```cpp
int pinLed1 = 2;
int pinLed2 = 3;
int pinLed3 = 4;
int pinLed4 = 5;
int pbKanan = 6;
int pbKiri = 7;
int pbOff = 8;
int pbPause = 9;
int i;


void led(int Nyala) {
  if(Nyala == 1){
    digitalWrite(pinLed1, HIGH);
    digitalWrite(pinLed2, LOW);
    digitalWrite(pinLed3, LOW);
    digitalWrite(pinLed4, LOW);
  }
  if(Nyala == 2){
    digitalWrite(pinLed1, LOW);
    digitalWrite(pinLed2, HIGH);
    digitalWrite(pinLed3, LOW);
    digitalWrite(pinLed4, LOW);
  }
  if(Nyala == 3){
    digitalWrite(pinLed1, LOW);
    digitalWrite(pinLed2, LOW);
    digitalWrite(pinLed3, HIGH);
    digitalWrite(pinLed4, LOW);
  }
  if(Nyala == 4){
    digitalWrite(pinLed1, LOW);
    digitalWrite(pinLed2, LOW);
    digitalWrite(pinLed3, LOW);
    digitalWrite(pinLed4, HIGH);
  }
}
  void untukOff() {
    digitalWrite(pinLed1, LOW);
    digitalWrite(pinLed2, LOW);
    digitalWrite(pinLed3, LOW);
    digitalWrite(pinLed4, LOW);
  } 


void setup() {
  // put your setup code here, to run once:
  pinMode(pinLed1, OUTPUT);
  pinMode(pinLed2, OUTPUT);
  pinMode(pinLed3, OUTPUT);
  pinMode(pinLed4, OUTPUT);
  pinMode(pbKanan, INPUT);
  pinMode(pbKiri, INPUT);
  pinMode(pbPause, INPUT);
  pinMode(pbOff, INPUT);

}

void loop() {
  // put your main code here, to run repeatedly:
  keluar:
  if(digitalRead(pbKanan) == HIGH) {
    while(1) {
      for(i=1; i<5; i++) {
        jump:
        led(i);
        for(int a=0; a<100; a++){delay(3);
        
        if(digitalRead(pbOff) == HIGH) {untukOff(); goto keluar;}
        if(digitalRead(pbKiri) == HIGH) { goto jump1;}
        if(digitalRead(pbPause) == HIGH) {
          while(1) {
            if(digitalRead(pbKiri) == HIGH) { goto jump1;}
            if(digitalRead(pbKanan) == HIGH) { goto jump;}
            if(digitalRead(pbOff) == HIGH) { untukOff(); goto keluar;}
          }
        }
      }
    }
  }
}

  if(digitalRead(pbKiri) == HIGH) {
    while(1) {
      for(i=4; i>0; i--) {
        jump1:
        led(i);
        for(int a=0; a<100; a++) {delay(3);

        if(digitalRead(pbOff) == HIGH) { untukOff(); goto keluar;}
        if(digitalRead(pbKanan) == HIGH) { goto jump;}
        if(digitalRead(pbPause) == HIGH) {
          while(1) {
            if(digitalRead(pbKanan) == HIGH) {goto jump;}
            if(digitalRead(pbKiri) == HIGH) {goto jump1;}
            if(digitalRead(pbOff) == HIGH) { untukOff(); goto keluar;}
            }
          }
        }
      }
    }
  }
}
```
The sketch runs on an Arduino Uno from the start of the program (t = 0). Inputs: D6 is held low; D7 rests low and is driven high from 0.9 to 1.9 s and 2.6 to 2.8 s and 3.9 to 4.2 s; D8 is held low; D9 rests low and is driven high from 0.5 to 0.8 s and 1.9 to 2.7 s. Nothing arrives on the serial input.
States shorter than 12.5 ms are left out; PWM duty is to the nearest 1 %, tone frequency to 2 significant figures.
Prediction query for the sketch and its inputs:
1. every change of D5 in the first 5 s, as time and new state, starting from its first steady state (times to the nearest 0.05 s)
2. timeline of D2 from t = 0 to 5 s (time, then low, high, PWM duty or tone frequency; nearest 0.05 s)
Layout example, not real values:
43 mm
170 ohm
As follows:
0 s low; 0.9 s high; 1.2 s low; 3 s high; 3.3 s low; 4.2 s high; 4.5 s low
0 s low; 1.8 s high; 3 s low; 3.9 s high; 4.2 s low
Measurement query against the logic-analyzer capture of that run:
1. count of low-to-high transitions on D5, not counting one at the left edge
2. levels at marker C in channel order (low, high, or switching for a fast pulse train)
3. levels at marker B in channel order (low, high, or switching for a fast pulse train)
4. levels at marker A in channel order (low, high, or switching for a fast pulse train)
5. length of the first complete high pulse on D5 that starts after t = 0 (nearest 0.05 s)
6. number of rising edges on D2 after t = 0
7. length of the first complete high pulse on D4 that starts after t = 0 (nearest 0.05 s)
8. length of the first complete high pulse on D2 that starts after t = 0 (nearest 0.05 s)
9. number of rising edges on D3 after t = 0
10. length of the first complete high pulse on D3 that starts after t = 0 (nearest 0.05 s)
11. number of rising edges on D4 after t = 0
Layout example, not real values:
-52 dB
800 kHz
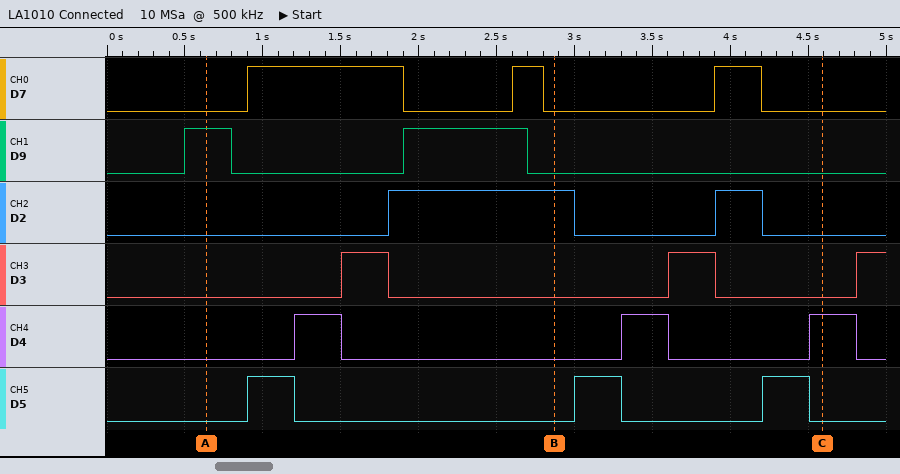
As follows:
3
D7 low, D9 low, D2 low, D3 low, D4 high, D5 low
D7 low, D9 low, D2 high, D3 low, D4 low, D5 low
D7 low, D9 high, D2 low, D3 low, D4 low, D5 low
0.30 s
2
0.30 s
1.20 s
3
0.30 s
3
